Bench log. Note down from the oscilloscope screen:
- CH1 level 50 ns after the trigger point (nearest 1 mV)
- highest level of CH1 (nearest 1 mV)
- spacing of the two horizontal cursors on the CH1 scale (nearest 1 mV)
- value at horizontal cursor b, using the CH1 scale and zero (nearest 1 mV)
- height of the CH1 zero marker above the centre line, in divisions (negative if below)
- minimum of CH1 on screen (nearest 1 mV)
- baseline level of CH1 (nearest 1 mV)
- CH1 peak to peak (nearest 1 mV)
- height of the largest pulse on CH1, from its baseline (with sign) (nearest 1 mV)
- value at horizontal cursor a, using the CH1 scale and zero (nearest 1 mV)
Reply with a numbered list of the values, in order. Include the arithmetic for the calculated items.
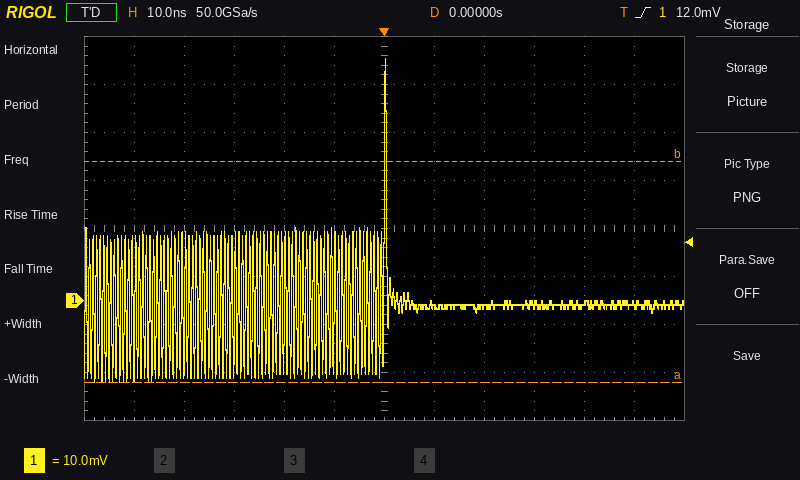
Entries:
1. -1 mV
2. 50 mV
3. 46 mV
4. 29 mV
5. -1.5 div
6. -17 mV
7. -1 mV
8. 50 mV − (-17 mV) = 67 mV
9. 50 mV − (-1 mV) = +51 mV
10. -17 mV
